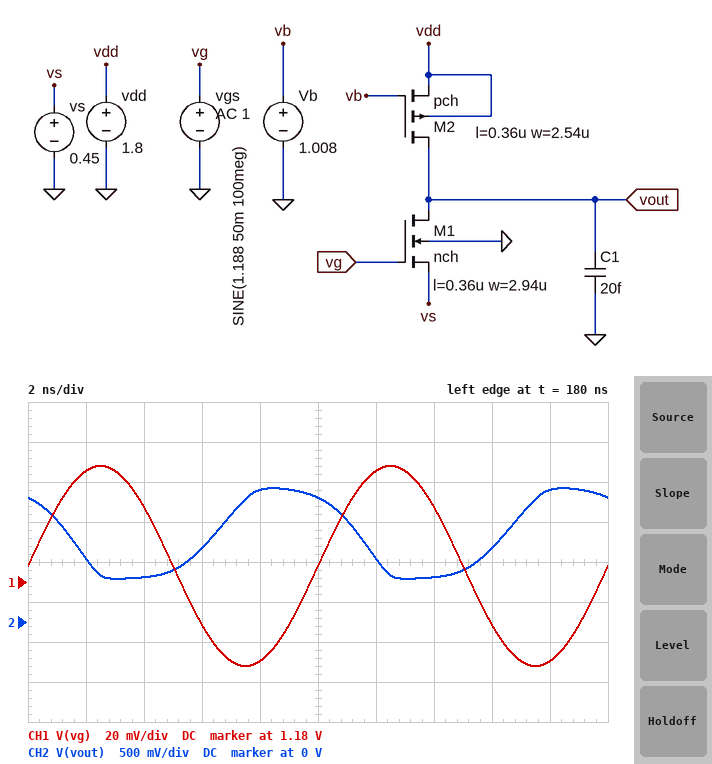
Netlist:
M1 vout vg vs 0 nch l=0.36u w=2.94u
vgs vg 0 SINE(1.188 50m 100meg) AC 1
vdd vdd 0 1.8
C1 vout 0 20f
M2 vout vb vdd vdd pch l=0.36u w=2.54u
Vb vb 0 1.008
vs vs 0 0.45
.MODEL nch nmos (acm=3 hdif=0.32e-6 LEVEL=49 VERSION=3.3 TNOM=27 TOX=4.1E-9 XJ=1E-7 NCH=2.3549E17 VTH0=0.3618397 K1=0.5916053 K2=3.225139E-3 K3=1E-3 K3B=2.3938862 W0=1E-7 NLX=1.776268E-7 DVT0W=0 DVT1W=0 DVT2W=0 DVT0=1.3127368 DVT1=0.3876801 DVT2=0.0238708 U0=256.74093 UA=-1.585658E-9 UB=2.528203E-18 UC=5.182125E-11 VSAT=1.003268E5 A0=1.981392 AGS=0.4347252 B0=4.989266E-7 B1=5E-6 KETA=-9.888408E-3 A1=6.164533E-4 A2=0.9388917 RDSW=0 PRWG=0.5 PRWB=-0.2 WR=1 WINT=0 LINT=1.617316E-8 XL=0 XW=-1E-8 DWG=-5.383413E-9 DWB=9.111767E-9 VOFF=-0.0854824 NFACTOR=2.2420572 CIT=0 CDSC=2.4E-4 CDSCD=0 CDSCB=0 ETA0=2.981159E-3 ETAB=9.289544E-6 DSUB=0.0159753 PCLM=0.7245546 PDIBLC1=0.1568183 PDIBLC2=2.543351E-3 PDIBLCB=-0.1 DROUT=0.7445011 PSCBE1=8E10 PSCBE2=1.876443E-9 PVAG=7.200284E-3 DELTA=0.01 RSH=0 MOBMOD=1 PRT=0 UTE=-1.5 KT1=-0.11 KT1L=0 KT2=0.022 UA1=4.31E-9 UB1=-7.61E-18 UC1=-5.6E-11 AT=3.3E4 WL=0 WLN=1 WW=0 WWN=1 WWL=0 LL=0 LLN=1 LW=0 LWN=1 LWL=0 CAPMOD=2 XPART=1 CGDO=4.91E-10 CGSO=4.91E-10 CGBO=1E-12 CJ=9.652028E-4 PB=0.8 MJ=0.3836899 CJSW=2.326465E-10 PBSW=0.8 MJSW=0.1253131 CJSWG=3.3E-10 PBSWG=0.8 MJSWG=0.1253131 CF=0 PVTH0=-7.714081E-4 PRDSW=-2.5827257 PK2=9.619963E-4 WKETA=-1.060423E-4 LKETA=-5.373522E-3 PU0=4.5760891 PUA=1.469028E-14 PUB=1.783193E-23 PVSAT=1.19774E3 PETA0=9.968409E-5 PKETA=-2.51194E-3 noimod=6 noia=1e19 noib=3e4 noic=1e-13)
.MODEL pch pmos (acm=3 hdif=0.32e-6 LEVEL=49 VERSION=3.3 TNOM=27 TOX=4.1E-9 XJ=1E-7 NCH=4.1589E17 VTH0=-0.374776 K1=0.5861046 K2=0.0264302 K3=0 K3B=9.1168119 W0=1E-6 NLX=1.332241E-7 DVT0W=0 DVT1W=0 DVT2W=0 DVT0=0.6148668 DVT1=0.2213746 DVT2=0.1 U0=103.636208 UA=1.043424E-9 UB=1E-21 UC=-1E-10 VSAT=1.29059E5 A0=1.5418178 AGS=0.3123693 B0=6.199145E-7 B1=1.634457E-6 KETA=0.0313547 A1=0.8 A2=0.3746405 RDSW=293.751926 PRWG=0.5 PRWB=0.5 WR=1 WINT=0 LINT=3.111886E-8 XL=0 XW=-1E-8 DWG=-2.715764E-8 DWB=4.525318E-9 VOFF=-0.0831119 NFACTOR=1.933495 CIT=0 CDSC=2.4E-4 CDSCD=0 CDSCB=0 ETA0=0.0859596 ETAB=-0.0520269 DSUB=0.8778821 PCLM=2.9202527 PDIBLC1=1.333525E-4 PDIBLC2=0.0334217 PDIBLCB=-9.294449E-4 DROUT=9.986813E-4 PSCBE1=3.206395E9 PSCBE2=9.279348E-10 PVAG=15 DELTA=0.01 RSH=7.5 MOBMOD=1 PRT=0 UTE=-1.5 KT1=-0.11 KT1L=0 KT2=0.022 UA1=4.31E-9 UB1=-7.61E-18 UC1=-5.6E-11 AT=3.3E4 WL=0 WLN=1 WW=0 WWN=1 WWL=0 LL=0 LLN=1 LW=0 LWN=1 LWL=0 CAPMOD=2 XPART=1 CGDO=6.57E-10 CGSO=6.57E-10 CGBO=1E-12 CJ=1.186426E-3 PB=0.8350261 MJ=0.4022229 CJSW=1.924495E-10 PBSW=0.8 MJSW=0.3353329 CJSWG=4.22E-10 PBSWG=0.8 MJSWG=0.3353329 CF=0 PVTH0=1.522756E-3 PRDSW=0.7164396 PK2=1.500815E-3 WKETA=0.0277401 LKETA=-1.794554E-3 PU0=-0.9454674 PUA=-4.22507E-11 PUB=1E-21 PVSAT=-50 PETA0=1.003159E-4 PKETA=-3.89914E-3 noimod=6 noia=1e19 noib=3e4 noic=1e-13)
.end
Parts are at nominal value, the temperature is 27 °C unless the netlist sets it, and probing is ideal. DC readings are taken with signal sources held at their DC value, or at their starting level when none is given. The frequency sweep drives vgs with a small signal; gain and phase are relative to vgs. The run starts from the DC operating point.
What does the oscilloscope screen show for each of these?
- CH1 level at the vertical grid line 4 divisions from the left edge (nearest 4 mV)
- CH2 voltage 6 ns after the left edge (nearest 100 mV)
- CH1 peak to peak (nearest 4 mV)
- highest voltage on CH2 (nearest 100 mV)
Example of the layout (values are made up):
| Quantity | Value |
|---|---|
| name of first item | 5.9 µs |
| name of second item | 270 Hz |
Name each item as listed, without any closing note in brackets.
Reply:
| Quantity | Value |
|---|---|
| CH1 level at the vertical grid line 4 divisions from the left edge | 1.140 V |
| CH2 voltage 6 ns after the left edge | 900 mV |
| CH1 peak to peak | 100 mV |
| highest voltage on CH2 | 1.7 V |
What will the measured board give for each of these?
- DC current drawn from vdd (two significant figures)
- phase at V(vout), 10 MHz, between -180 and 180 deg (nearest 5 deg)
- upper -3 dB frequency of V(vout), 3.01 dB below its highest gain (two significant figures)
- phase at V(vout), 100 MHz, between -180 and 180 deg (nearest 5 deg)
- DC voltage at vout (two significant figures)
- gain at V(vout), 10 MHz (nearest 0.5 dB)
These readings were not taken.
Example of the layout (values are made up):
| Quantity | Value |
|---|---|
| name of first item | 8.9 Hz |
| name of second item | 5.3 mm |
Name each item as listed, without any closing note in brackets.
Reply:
| Quantity | Value |
|---|---|
| DC current drawn from vdd | 29 µA |
| phase at V(vout), 10 MHz, between -180 and 180 deg | 170 deg |
| upper -3 dB frequency of V(vout), 3.01 dB below its highest gain | 47 MHz |
| phase at V(vout), 100 MHz, between -180 and 180 deg | 115 deg |
| DC voltage at vout | 1.2 V |
| gain at V(vout), 10 MHz | 32.0 dB |
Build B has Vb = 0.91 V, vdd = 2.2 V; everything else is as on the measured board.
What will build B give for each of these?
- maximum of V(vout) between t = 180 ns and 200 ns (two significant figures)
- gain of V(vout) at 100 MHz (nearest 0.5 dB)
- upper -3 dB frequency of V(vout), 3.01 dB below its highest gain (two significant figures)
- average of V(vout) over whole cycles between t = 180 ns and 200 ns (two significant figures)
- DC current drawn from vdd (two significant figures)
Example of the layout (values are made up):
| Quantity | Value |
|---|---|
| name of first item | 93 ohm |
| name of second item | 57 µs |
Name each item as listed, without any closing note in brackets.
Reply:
| Quantity | Value |
|---|---|
| maximum of V(vout) between t = 180 ns and 200 ns | 2.2 V |
| gain of V(vout) at 100 MHz | 0.5 dB |
| upper -3 dB frequency of V(vout), 3.01 dB below its highest gain | 1.5 GHz |
| average of V(vout) over whole cycles between t = 180 ns and 200 ns | 2.1 V |
| DC current drawn from vdd | 33 µA |
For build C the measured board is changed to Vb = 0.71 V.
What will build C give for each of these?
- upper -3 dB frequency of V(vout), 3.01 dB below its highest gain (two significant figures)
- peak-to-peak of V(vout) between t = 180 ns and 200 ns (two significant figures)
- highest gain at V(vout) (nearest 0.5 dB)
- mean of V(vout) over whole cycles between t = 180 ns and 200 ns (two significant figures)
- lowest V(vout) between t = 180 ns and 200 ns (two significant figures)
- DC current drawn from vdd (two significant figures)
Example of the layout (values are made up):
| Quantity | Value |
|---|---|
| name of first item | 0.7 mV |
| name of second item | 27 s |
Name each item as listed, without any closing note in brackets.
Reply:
| Quantity | Value |
|---|---|
| upper -3 dB frequency of V(vout), 3.01 dB below its highest gain | 1.1 GHz |
| peak-to-peak of V(vout) between t = 180 ns and 200 ns | 140 mV |
| highest gain at V(vout) | 3.0 dB |
| mean of V(vout) over whole cycles between t = 180 ns and 200 ns | 1.7 V |
| lowest V(vout) between t = 180 ns and 200 ns | 1.6 V |
| DC current drawn from vdd | 31 µA |
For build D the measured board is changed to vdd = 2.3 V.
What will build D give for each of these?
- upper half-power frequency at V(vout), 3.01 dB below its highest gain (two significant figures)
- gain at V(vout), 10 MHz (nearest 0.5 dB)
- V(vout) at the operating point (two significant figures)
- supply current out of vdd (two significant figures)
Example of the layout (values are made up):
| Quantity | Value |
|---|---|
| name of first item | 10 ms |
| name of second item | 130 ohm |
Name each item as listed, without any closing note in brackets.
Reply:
| Quantity | Value |
|---|---|
| upper half-power frequency at V(vout), 3.01 dB below its highest gain | 1.5 GHz |
| gain at V(vout), 10 MHz | 0.5 dB |
| V(vout) at the operating point | 2.2 V |
| supply current out of vdd | 33 µA |
